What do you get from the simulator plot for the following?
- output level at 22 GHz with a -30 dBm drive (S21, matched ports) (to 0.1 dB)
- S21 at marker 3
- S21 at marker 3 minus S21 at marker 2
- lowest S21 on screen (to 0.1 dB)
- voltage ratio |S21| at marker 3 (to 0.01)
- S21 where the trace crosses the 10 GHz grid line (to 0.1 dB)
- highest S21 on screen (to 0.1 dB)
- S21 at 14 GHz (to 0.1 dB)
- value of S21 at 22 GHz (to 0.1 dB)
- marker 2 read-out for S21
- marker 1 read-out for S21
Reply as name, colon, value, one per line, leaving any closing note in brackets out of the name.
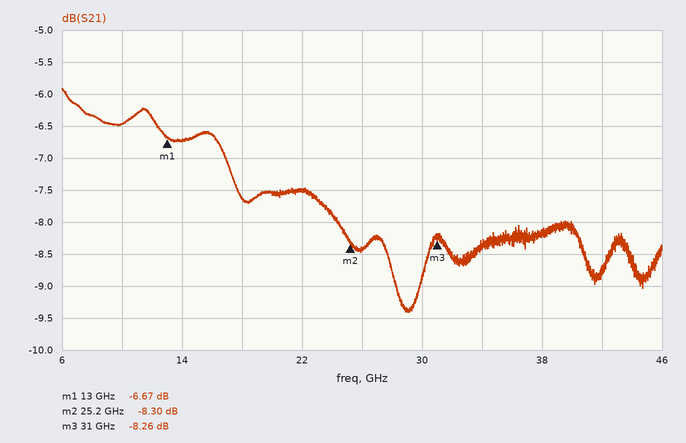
output level at 22 GHz with a -30 dBm drive (S21, matched ports): -37.5 dBm
S21 at marker 3: -8.26 dB
S21 at marker 3 minus S21 at marker 2: 0.04 dB
lowest S21 on screen: -9.4 dB
voltage ratio |S21| at marker 3: 0.39
S21 where the trace crosses the 10 GHz grid line: -6.5 dB
highest S21 on screen: -5.9 dB
S21 at 14 GHz: -6.7 dB
value of S21 at 22 GHz: -7.5 dB
marker 2 read-out for S21: -8.30 dB
marker 1 read-out for S21: -6.67 dB
